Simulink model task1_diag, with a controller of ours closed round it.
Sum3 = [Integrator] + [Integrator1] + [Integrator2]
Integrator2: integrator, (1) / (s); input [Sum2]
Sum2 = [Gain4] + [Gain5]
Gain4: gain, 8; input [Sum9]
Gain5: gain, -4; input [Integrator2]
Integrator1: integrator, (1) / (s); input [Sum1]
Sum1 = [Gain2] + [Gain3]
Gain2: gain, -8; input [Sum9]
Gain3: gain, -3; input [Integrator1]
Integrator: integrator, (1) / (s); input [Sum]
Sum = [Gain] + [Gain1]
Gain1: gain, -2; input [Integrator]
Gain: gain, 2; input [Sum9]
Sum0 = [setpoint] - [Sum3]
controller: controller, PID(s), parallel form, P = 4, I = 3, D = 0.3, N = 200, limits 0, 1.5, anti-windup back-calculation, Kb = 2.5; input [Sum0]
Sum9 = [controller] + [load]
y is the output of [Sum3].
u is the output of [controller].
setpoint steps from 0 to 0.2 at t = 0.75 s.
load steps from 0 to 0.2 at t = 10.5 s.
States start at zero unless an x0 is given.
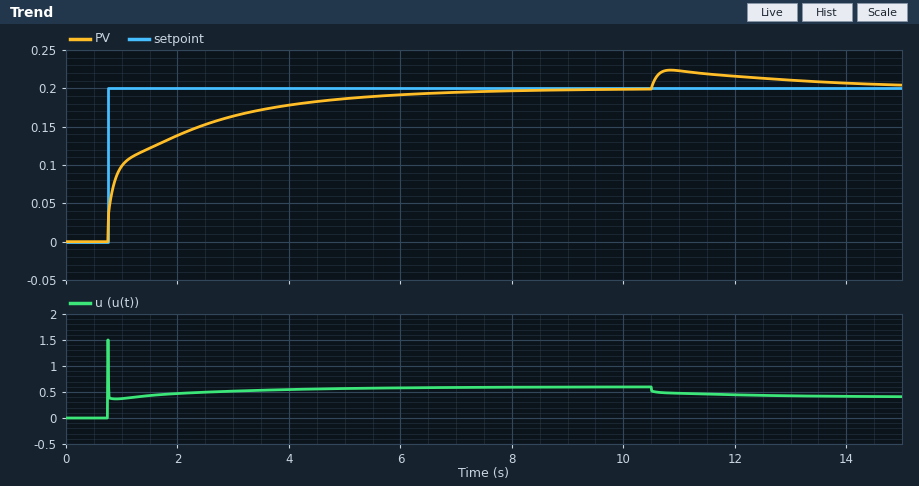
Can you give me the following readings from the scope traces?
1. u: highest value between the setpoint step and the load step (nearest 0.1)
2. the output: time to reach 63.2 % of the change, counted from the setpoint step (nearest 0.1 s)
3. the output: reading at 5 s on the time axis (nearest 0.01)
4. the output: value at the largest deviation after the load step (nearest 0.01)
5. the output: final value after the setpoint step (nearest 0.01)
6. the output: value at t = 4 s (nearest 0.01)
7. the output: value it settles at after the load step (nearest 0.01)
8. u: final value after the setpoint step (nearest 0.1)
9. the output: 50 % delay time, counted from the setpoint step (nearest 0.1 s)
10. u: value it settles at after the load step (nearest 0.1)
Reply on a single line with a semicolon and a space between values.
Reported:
1.5; 0.9 s; 0.19; 0.22; 0.20; 0.18; 0.20; 0.6; 0.3 s; 0.4
